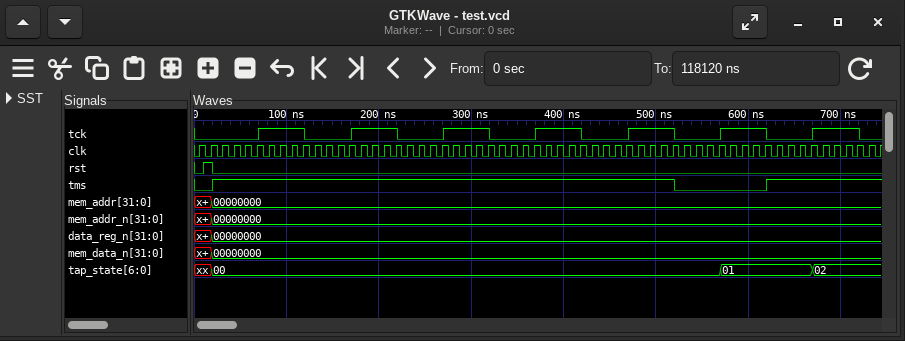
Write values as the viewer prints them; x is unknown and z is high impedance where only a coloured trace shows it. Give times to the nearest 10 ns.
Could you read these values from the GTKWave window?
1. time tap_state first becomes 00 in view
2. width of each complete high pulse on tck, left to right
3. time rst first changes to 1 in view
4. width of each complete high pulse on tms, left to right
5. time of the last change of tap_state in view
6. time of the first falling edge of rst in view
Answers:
20 ns
50 ns, 50 ns, 50 ns, 50 ns, 50 ns, 50 ns, 50 ns
10 ns
500 ns
670 ns
20 ns
